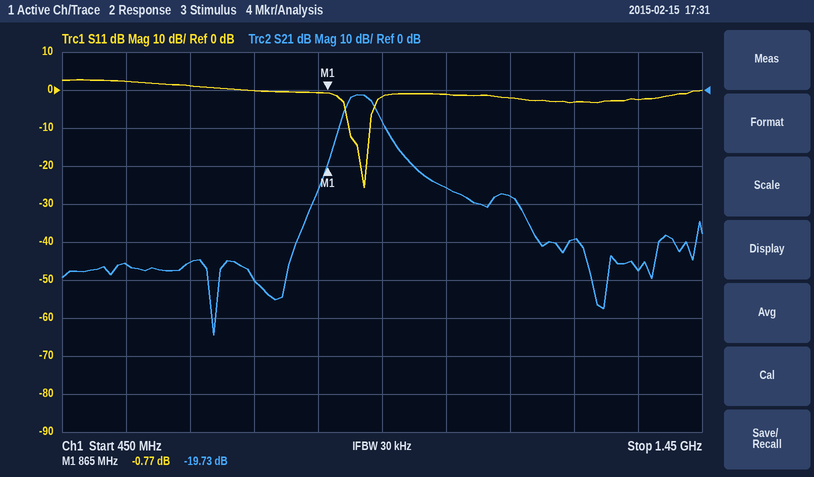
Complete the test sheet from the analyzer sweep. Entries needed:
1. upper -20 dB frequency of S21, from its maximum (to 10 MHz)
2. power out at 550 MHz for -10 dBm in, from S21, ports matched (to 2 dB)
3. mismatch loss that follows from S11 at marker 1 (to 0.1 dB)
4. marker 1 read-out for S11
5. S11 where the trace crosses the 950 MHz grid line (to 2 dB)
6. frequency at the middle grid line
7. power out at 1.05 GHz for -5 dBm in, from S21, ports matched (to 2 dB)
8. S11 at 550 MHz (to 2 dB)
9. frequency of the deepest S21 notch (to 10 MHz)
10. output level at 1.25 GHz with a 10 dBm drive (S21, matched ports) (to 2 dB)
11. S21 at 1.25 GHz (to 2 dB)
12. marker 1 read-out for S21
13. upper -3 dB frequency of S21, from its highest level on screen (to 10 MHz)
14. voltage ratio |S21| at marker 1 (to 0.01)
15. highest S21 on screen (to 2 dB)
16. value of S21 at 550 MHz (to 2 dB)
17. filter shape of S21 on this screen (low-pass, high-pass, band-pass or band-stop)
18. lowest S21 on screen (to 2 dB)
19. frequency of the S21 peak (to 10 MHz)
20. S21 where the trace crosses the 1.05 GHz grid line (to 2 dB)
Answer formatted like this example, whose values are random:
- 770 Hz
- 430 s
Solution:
- 1.01 GHz
- -56 dBm
- 7.9 dB
- -0.77 dB
- -2 dB
- 950 MHz
- -30 dBm
- 2 dB
- 690 MHz
- -30 dBm
- -40 dB
- -19.73 dB
- 940 MHz
- 0.10
- -2 dB
- -46 dB
- band-pass
- -64 dB
- 910 MHz
- -26 dB
